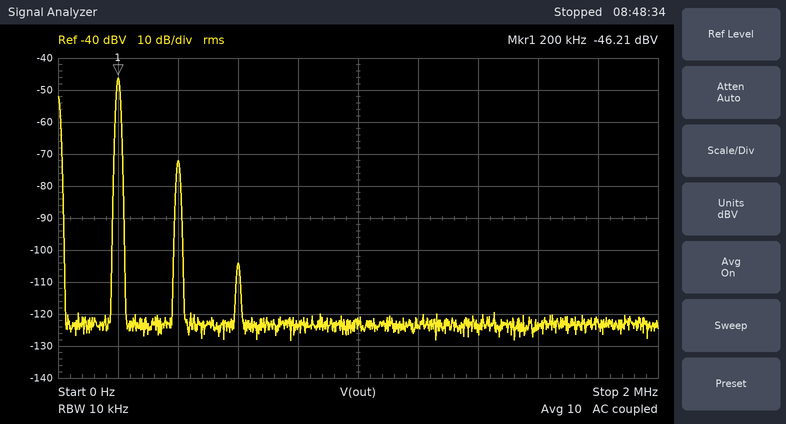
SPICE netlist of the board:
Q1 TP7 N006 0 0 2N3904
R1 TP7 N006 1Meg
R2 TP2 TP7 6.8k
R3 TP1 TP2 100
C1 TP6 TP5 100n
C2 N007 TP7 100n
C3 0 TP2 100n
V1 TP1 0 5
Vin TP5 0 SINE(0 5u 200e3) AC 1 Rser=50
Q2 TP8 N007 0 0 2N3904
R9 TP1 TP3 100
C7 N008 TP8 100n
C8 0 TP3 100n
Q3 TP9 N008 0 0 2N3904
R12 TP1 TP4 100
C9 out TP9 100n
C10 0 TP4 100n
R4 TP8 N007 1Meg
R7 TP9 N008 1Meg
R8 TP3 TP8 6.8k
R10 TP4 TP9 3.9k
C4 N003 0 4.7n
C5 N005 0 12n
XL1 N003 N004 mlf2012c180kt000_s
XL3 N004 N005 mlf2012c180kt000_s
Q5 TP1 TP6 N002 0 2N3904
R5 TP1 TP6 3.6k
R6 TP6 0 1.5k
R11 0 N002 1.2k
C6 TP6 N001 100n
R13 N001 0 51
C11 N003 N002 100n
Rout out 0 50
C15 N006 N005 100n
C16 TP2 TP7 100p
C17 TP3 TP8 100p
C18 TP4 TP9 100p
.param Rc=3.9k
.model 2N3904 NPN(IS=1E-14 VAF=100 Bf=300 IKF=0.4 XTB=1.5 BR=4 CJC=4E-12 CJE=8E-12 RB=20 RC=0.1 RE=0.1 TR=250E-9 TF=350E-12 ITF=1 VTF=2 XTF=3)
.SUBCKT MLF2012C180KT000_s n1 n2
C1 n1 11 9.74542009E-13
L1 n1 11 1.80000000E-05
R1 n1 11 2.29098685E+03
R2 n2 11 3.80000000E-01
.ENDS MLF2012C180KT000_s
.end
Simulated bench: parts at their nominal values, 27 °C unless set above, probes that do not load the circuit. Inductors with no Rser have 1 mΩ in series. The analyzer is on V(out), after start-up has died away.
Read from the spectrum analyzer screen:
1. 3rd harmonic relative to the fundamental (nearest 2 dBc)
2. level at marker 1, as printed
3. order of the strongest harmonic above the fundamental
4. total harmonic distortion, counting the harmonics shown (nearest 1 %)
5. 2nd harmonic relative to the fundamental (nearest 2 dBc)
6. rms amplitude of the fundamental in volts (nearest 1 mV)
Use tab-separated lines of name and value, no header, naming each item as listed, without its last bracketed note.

3rd harmonic relative to the fundamental	-58 dBc
level at marker 1, as printed	-46.21 dBV
order of the strongest harmonic above the fundamental	2
total harmonic distortion, counting the harmonics shown	5 %
2nd harmonic relative to the fundamental	-26 dBc
rms amplitude of the fundamental in volts	5 mV
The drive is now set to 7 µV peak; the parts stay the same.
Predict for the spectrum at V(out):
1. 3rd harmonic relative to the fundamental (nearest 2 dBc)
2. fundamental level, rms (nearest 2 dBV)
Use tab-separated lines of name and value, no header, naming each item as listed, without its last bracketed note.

3rd harmonic relative to the fundamental	-52 dBc
fundamental level, rms	-44 dBV
